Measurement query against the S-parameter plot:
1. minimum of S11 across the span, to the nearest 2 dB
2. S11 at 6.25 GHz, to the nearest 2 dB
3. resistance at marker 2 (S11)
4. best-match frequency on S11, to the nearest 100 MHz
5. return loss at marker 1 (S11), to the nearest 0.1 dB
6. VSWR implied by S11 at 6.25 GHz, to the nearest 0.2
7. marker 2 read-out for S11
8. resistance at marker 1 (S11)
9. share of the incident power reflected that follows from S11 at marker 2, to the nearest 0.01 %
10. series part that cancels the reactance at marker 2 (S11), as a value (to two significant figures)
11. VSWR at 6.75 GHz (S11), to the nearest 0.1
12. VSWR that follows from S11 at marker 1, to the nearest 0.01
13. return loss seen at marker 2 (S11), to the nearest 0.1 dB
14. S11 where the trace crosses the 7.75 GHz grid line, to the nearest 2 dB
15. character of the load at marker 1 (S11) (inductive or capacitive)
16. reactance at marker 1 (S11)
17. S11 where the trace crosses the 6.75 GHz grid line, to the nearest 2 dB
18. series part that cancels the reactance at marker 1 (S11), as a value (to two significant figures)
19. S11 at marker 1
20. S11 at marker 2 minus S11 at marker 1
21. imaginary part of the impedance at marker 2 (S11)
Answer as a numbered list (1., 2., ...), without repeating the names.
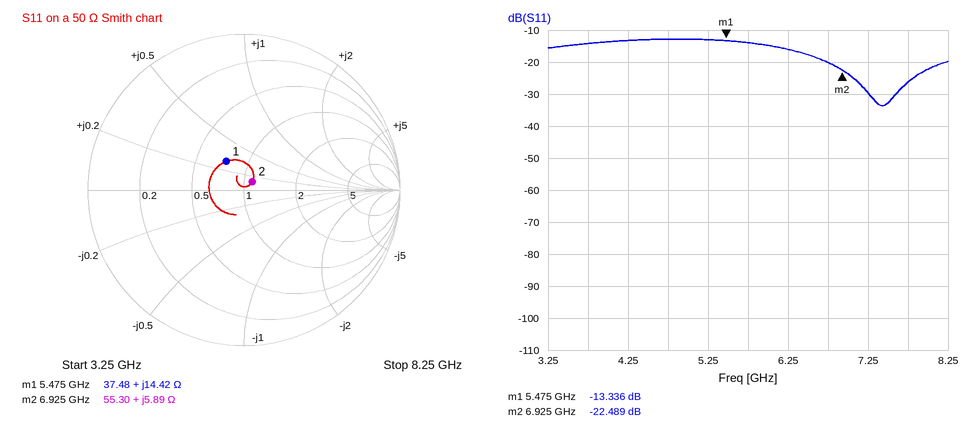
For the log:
1. -34 dB
2. -16 dB
3. 55.30 Ω
4. 7.4 GHz
5. 13.3 dB
6. 1.4
7. -22.489 dB
8. 37.48 Ω
9. 0.56 %
10. 3.9 pF
11. 1.2
12. 1.55
13. 22.5 dB
14. -26 dB
15. inductive
16. +14.42 Ω
17. -20 dB
18. 2.0 pF
19. -13.336 dB
20. -9.153 dB
21. +5.89 Ω
